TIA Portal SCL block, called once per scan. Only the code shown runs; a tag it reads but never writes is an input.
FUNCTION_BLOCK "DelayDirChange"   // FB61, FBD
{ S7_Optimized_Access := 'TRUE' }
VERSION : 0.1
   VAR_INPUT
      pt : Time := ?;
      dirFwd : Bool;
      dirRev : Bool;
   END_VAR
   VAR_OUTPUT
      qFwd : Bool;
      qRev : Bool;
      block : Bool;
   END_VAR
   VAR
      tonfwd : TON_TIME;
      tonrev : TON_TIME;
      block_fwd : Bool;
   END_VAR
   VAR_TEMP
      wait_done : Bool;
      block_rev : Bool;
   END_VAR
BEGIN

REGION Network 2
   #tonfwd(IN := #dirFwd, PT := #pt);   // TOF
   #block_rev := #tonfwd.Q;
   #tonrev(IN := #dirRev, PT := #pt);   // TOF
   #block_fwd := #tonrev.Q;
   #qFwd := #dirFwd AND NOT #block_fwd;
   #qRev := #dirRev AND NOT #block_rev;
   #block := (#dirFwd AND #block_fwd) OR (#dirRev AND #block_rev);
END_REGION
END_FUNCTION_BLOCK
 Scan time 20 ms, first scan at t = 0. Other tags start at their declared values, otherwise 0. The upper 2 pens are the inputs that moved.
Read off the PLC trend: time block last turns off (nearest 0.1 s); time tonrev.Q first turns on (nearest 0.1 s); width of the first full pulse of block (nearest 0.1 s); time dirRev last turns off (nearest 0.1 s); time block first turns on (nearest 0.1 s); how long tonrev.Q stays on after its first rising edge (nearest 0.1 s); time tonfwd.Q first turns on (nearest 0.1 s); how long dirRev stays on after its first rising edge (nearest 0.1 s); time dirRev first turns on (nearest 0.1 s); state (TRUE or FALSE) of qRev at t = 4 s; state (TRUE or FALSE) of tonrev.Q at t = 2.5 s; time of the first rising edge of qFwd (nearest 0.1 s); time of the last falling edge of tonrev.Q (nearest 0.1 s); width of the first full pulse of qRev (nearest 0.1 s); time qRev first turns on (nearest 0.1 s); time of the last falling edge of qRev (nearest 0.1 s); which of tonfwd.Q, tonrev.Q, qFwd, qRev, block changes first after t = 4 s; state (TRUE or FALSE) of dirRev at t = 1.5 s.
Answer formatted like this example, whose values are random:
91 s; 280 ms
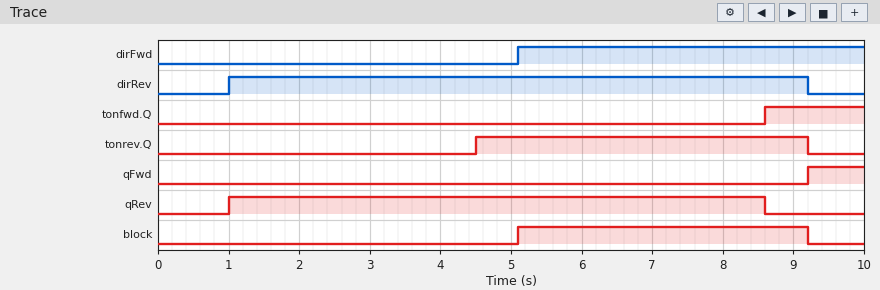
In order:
9.2 s; 4.5 s; 4.1 s; 9.2 s; 5.1 s; 4.7 s; 8.6 s; 8.2 s; 1.0 s; TRUE; FALSE; 9.2 s; 9.2 s; 7.6 s; 1.0 s; 8.6 s; tonrev.Q; TRUE
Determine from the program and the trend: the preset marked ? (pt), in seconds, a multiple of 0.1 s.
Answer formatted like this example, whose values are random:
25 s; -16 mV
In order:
3.5 s
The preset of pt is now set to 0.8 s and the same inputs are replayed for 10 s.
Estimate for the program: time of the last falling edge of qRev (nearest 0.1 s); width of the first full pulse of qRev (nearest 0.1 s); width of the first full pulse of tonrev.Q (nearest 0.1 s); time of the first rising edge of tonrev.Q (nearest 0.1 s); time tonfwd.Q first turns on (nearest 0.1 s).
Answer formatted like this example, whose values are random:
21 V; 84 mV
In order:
5.9 s; 4.9 s; 7.4 s; 1.8 s; 5.9 s
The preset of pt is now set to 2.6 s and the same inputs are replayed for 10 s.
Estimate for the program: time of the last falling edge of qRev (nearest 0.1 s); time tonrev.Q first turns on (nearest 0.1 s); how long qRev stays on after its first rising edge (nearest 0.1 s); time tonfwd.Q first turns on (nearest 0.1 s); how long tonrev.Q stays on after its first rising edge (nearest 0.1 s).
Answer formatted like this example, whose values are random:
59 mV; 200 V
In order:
7.7 s; 3.6 s; 6.7 s; 7.7 s; 5.6 s
